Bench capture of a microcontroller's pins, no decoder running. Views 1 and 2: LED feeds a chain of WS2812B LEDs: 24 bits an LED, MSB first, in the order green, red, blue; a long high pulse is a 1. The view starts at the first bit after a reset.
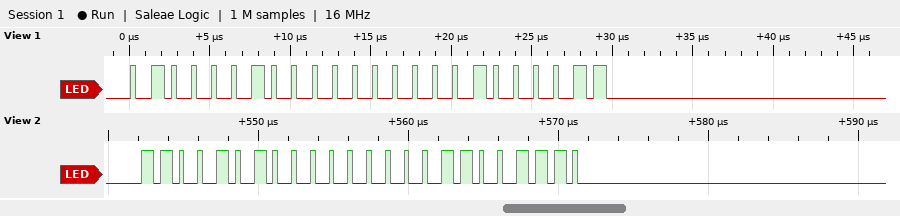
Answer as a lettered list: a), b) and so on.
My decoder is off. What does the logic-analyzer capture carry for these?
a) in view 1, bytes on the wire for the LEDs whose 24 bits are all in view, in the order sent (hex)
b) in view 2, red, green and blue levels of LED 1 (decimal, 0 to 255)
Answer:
a) 42 00 43
b) 0, 202, 206
